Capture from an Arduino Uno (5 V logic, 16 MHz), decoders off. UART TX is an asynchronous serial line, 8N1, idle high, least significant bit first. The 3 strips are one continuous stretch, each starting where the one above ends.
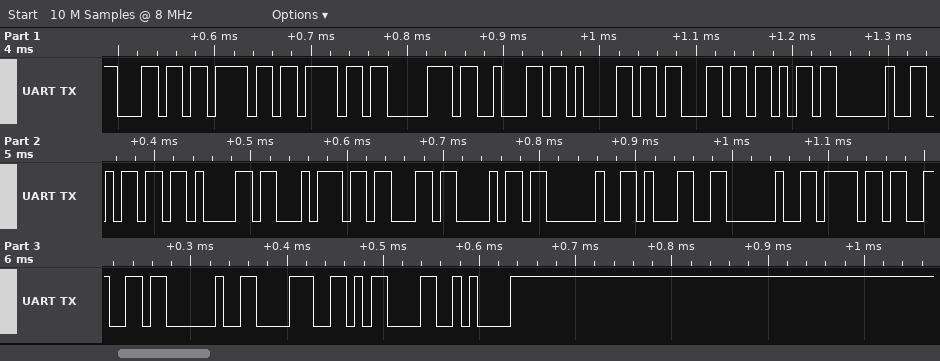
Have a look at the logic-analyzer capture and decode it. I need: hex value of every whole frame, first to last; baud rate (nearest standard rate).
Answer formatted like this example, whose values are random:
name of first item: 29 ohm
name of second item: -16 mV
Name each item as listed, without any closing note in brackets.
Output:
hex value of every whole frame, first to last: 0x6C 0x6F 0x6F 0x70 0x62 0x61 0x63 0x6B 0x20 0x6D 0x61 0x74 0x63 0x68 0x20 0x31 0x20 0x6F 0x66 0x20 0x38 0x0D 0x0A
baud rate: 115200 baud
